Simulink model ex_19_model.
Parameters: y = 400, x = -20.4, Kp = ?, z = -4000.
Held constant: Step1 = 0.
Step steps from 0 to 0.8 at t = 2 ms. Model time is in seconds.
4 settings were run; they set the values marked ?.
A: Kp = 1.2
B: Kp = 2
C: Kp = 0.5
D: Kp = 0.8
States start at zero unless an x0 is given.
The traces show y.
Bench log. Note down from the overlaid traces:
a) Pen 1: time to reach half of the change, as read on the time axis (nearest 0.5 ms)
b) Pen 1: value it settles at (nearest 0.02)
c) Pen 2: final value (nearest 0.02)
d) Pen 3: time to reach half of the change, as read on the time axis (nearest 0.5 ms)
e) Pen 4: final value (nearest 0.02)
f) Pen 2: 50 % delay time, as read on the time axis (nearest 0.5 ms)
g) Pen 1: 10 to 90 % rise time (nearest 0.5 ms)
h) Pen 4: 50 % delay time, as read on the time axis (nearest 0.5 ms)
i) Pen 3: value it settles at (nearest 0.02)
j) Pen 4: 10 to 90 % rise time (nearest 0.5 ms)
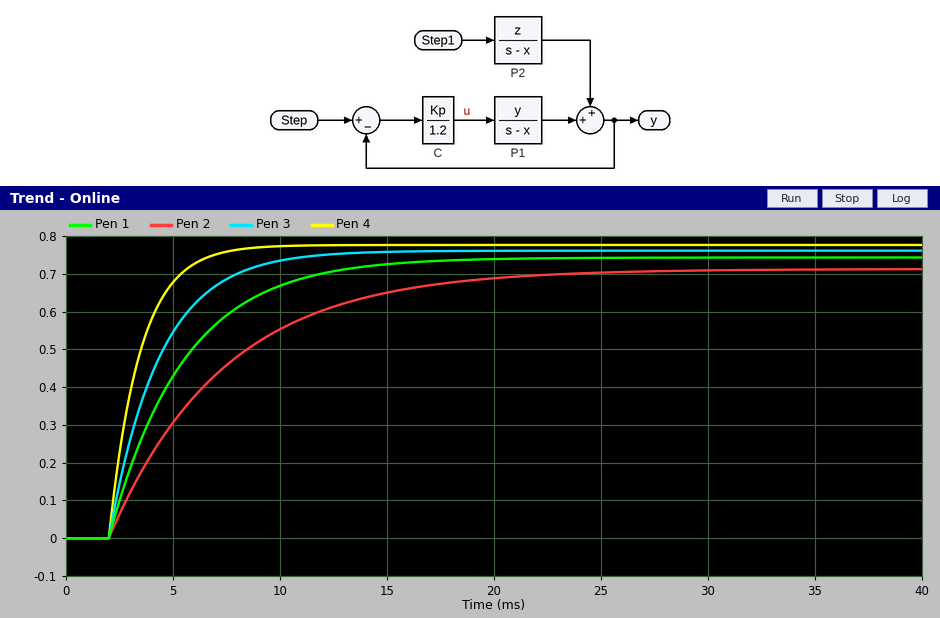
4.5 ms
0.74
0.72
3.5 ms
0.78
5.5 ms
7.5 ms
3.0 ms
0.76
3.0 ms
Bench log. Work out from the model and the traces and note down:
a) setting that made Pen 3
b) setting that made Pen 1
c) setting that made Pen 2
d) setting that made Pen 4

A
D
C
B
